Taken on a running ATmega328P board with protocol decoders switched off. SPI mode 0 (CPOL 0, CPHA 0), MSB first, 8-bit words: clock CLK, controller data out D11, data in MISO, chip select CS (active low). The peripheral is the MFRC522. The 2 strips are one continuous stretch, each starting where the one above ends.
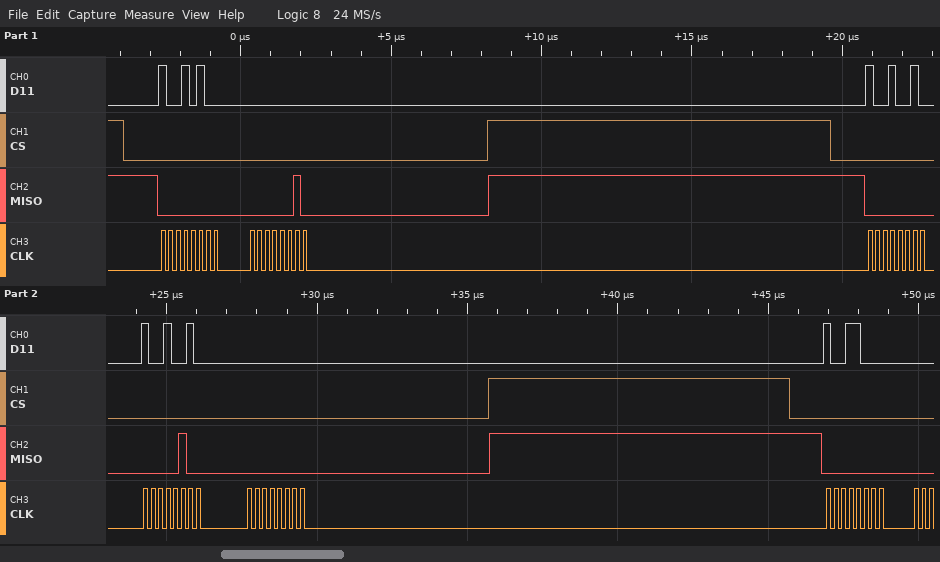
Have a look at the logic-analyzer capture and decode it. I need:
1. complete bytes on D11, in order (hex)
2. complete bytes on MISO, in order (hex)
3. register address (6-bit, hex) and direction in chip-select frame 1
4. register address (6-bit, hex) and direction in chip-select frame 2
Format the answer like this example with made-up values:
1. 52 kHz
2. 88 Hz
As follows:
1. 94 00 92 92 00 98
2. 00 02 00 04 00 00
3. 0x0A read
4. 0x09 read
